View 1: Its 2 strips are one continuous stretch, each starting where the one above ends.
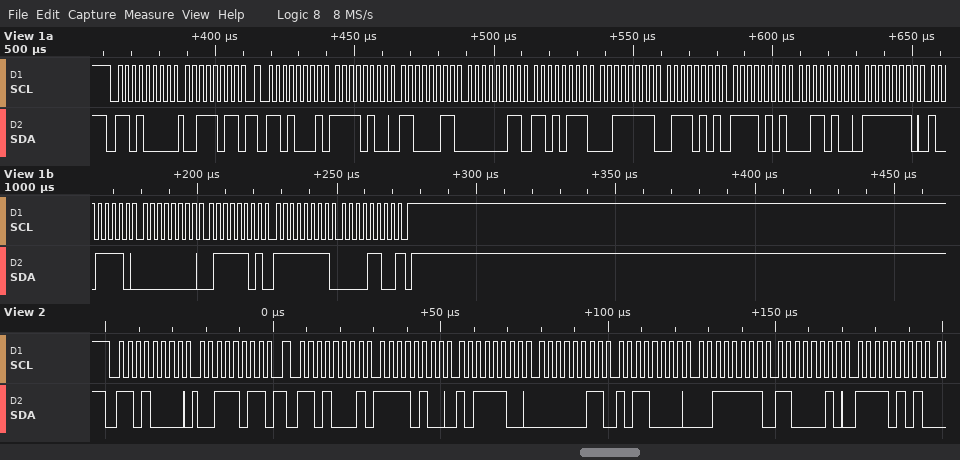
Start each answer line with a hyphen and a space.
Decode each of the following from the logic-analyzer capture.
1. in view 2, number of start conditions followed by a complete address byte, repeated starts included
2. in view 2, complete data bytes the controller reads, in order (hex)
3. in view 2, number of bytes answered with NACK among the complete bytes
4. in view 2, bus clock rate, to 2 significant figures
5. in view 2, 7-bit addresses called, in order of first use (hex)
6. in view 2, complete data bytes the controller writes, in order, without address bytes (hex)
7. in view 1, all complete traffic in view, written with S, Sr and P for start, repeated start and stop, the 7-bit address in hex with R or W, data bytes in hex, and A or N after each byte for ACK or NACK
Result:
- 2
- F4 BC 03 B0 3F C2 F5
- 0
- 400 kHz
- 0x68
- 3B
- S 68W A 3B A Sr 68R A F4 A C3 A 03 A D7 A 3F A 75 A F5 A 34 A FE A 9E A 00 A 7D A FF A 0C N P
